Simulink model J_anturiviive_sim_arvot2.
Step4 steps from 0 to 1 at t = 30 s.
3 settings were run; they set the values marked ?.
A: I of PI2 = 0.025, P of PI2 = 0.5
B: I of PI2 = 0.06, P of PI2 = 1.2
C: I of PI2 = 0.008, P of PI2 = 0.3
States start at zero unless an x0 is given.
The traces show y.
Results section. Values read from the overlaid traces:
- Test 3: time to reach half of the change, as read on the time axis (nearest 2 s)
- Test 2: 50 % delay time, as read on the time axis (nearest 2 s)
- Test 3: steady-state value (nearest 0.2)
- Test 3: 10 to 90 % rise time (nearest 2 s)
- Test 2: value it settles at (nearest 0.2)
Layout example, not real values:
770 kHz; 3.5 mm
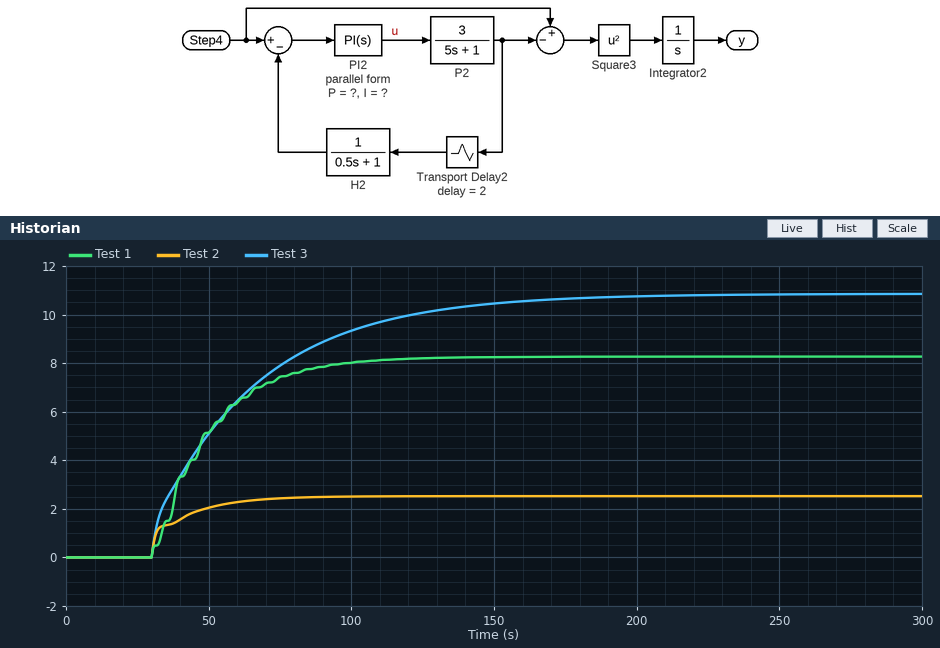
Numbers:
52 s; 34 s; 10.8; 82 s; 2.6
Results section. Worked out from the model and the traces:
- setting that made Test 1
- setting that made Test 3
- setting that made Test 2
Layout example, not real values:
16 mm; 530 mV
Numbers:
B; C; A
